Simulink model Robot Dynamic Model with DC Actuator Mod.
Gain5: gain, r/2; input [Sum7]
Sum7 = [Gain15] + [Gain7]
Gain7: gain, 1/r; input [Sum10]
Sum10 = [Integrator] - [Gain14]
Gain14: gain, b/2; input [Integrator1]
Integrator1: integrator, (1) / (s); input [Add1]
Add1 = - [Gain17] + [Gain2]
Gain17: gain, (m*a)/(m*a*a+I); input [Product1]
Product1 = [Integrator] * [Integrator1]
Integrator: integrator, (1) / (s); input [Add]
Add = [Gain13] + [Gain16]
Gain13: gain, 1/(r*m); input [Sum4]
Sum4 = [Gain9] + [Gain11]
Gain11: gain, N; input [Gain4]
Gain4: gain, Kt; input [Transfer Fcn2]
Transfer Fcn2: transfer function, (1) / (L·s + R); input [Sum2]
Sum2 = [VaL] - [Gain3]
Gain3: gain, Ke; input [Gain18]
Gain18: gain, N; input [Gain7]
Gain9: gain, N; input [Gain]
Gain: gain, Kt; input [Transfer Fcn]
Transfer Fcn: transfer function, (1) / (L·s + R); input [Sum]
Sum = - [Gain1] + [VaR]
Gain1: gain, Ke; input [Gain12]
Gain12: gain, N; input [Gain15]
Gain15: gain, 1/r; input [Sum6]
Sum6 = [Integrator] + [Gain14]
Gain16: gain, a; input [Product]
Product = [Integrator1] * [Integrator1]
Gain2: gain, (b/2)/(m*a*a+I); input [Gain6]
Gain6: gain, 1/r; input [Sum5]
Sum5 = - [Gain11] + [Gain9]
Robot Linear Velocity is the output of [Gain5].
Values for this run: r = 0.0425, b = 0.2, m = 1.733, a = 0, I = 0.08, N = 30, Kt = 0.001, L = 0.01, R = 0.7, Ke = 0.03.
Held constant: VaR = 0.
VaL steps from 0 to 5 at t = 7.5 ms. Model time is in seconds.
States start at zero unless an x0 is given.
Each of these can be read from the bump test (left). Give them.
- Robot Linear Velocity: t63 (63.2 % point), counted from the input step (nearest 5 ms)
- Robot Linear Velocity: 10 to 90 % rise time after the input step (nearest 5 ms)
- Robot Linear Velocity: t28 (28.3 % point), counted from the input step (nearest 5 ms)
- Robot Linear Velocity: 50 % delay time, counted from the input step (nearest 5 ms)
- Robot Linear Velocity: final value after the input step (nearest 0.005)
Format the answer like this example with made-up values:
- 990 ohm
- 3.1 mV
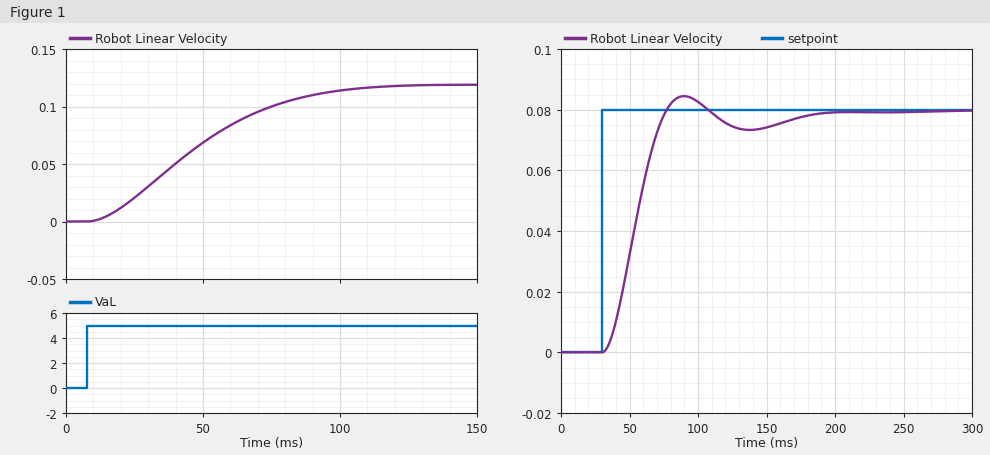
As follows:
- 45 ms
- 65 ms
- 25 ms
- 35 ms
- 0.120
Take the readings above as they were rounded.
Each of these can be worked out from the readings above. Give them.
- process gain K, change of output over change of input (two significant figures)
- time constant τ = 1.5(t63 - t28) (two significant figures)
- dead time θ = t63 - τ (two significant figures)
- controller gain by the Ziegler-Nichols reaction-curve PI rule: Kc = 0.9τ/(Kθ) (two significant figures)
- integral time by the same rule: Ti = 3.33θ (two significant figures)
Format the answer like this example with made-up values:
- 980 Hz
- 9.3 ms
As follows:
- 0.024
- 30 ms
- 15 ms
- 75
- 50 ms
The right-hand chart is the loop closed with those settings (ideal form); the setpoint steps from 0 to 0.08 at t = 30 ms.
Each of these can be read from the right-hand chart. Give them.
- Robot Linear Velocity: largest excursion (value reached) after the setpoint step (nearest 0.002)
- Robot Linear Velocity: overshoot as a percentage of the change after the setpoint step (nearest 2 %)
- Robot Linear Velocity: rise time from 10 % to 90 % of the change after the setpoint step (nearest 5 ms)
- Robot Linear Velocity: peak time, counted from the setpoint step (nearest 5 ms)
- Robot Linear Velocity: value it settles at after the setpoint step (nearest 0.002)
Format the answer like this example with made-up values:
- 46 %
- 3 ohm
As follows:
- 0.084
- 6 %
- 30 ms
- 60 ms
- 0.080
